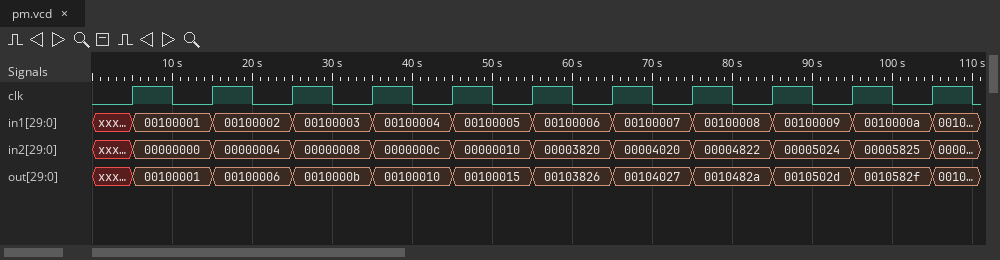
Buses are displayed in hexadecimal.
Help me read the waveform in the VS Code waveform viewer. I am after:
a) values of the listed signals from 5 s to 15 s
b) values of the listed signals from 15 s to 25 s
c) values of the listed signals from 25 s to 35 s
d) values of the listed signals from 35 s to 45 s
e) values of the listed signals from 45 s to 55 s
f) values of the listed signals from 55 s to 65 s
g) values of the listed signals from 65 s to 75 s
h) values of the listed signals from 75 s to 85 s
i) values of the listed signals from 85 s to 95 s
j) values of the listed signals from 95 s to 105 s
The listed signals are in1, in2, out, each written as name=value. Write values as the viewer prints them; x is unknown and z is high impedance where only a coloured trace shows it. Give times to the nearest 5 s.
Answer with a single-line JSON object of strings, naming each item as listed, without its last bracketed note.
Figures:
{"values of the listed signals from 5 s to 15 s": "in1=00100001, in2=00000000, out=00100001", "values of the listed signals from 15 s to 25 s": "in1=00100002, in2=00000004, out=00100006", "values of the listed signals from 25 s to 35 s": "in1=00100003, in2=00000008, out=0010000b", "values of the listed signals from 35 s to 45 s": "in1=00100004, in2=0000000c, out=00100010", "values of the listed signals from 45 s to 55 s": "in1=00100005, in2=00000010, out=00100015", "values of the listed signals from 55 s to 65 s": "in1=00100006, in2=00003820, out=00103826", "values of the listed signals from 65 s to 75 s": "in1=00100007, in2=00004020, out=00104027", "values of the listed signals from 75 s to 85 s": "in1=00100008, in2=00004822, out=0010482a", "values of the listed signals from 85 s to 95 s": "in1=00100009, in2=00005024, out=0010502d", "values of the listed signals from 95 s to 105 s": "in1=0010000a, in2=00005825, out=0010582f"}
